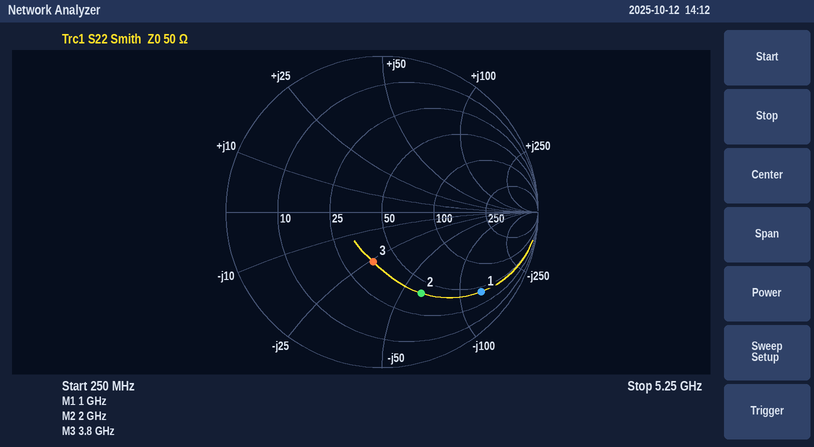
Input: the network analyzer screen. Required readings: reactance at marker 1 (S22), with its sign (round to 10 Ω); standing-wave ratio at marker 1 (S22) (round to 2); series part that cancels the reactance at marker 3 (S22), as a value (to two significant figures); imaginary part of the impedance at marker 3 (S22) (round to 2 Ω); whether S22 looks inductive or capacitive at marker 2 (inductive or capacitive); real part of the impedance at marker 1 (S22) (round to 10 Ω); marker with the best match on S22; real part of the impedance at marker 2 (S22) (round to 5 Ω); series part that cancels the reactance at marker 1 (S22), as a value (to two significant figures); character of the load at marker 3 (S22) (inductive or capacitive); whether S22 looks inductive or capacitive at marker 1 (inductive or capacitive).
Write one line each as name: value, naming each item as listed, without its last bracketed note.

reactance at marker 1 (S22), with its sign: -130 Ω
standing-wave ratio at marker 1 (S22): 10
series part that cancels the reactance at marker 3 (S22), as a value: 1.1 nH
imaginary part of the impedance at marker 3 (S22): -26 Ω
whether S22 looks inductive or capacitive at marker 2: capacitive
real part of the impedance at marker 1 (S22): 40 Ω
marker with the best match on S22: marker 3
real part of the impedance at marker 2 (S22): 40 Ω
series part that cancels the reactance at marker 1 (S22), as a value: 21 nH
character of the load at marker 3 (S22): capacitive
whether S22 looks inductive or capacitive at marker 1: capacitive
